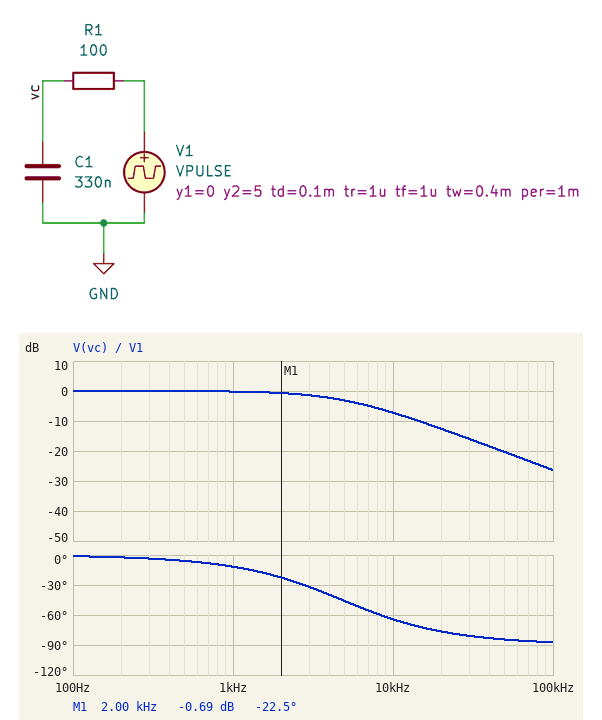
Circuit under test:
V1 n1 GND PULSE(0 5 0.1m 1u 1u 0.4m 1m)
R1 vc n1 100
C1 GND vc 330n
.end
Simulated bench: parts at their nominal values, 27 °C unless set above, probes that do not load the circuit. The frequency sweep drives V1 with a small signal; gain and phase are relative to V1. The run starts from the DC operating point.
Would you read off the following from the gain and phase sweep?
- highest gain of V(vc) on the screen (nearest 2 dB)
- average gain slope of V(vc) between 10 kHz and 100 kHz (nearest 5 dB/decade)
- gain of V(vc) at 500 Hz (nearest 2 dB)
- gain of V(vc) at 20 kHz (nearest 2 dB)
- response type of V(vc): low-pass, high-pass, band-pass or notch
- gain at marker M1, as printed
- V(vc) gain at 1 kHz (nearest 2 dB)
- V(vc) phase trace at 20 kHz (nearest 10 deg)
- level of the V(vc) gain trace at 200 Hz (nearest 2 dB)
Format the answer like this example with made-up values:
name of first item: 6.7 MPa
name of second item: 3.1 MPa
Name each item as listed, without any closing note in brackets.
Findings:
highest gain of V(vc) on the screen: 0 dB
average gain slope of V(vc) between 10 kHz and 100 kHz: -20 dB/decade
gain of V(vc) at 500 Hz: 0 dB
gain of V(vc) at 20 kHz: -12 dB
response type of V(vc): low-pass, high-pass, band-pass or notch: low-pass
gain at marker M1, as printed: -0.69 dB
V(vc) gain at 1 kHz: 0 dB
V(vc) phase trace at 20 kHz: -80 deg
level of the V(vc) gain trace at 200 Hz: 0 dB
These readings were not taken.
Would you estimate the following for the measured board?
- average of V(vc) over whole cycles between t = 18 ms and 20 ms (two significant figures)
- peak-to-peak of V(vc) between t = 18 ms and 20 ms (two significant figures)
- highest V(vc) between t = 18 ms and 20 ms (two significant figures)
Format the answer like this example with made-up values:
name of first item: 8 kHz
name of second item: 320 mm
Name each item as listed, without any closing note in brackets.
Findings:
average of V(vc) over whole cycles between t = 18 ms and 20 ms: 2.0 V
peak-to-peak of V(vc) between t = 18 ms and 20 ms: 5.0 V
highest V(vc) between t = 18 ms and 20 ms: 5.0 V
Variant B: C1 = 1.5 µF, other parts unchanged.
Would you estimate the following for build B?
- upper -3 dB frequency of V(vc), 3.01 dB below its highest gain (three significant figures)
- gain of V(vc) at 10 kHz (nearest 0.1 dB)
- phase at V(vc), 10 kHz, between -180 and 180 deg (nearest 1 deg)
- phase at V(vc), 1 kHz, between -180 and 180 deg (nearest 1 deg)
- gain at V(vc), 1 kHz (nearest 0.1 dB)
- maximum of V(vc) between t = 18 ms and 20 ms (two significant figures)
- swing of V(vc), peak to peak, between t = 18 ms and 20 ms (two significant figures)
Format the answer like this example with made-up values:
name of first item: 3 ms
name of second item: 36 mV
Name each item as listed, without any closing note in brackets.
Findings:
upper -3 dB frequency of V(vc), 3.01 dB below its highest gain: 1.06 kHz
gain of V(vc) at 10 kHz: -19.5 dB
phase at V(vc), 10 kHz, between -180 and 180 deg: -84 deg
phase at V(vc), 1 kHz, between -180 and 180 deg: -43 deg
gain at V(vc), 1 kHz: -2.8 dB
maximum of V(vc) between t = 18 ms and 20 ms: 4.7 V
swing of V(vc), peak to peak, between t = 18 ms and 20 ms: 4.6 V
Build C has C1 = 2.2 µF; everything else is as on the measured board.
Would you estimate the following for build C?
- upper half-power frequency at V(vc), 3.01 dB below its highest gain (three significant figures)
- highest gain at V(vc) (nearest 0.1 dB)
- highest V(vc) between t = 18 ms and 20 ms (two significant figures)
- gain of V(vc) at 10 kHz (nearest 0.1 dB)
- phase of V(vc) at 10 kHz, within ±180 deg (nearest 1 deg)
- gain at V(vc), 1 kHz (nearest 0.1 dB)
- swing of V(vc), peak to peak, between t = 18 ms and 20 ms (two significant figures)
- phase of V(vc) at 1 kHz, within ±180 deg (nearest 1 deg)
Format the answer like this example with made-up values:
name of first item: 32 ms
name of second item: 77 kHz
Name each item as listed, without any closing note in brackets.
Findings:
upper half-power frequency at V(vc), 3.01 dB below its highest gain: 723 Hz
highest gain at V(vc): 0 dB
highest V(vc) between t = 18 ms and 20 ms: 4.2 V
gain of V(vc) at 10 kHz: -22.8 dB
phase of V(vc) at 10 kHz, within ±180 deg: -86 deg
gain at V(vc), 1 kHz: -4.6 dB
swing of V(vc), peak to peak, between t = 18 ms and 20 ms: 4.0 V
phase of V(vc) at 1 kHz, within ±180 deg: -54 deg
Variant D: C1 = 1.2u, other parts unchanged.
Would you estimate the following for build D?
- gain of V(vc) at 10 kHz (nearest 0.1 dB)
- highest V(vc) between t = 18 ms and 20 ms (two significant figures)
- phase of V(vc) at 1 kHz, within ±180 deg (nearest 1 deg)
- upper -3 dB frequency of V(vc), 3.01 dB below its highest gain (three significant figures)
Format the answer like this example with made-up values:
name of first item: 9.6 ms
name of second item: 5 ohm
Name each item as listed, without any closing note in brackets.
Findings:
gain of V(vc) at 10 kHz: -17.6 dB
highest V(vc) between t = 18 ms and 20 ms: 4.8 V
phase of V(vc) at 1 kHz, within ±180 deg: -37 deg
upper -3 dB frequency of V(vc), 3.01 dB below its highest gain: 1.33 kHz
